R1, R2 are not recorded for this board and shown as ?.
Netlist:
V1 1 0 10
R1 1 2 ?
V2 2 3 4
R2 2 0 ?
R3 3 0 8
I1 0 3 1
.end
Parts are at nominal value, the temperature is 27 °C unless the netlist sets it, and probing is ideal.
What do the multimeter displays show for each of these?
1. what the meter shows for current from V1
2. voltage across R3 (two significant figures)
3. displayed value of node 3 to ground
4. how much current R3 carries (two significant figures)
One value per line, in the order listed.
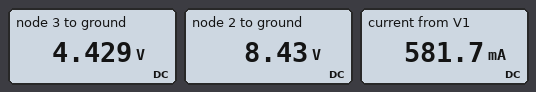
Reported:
581.7 mA
4.4 V
4.429 V
550 mA
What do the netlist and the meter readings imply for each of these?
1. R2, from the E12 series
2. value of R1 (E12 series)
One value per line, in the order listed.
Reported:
8.2 Ω
2.7 Ω
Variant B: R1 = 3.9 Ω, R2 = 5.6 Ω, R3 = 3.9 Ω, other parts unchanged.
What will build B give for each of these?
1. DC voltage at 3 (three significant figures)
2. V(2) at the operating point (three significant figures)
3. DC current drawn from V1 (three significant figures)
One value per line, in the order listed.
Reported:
2.64 V
6.64 V
862 mA
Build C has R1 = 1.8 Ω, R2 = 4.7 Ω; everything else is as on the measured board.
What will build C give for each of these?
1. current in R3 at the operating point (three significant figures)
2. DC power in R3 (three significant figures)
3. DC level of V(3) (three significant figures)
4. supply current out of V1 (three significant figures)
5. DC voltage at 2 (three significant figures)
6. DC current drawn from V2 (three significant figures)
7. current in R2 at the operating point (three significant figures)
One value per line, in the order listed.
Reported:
487 mA
1.90 W
3.90 V
1.17 A
7.90 V
513 mA
1.68 A
